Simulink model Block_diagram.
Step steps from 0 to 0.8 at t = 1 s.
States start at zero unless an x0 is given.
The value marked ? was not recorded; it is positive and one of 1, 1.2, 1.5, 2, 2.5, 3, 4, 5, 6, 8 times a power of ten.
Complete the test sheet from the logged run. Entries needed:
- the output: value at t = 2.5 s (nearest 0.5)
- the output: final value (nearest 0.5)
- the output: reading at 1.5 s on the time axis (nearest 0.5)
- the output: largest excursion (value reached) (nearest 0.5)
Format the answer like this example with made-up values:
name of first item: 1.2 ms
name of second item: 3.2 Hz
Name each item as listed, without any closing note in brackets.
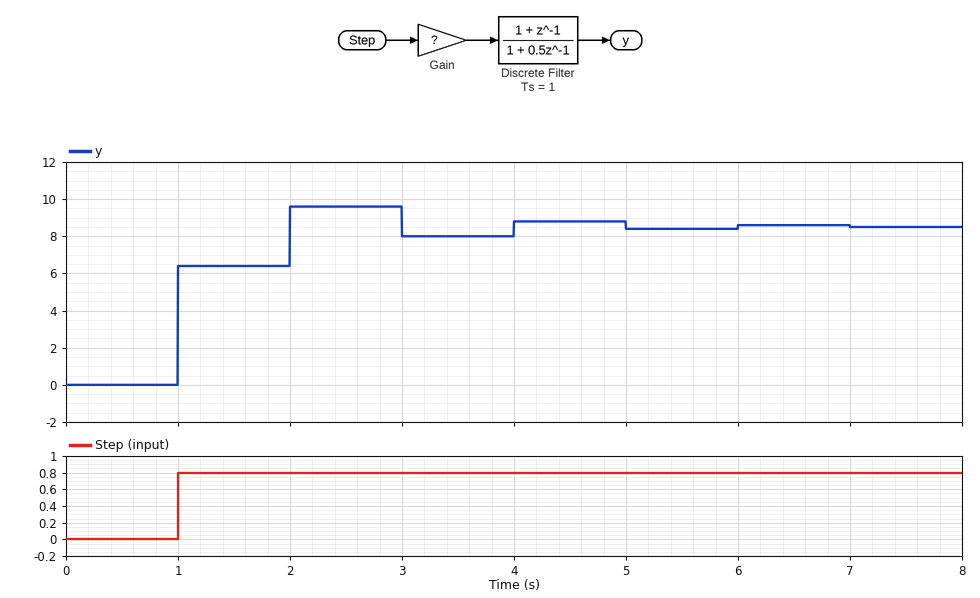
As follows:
the output: value at t = 2.5 s: 9.5
the output: final value: 8.5
the output: reading at 1.5 s on the time axis: 6.5
the output: largest excursion (value reached): 9.5
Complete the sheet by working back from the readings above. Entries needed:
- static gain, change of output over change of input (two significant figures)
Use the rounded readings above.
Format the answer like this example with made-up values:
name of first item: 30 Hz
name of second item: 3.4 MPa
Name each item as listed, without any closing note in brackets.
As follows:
static gain, change of output over change of input: 11
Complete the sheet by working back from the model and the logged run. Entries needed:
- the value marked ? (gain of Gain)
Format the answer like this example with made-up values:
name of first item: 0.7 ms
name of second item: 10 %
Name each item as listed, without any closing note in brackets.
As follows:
the value marked ?: 8
